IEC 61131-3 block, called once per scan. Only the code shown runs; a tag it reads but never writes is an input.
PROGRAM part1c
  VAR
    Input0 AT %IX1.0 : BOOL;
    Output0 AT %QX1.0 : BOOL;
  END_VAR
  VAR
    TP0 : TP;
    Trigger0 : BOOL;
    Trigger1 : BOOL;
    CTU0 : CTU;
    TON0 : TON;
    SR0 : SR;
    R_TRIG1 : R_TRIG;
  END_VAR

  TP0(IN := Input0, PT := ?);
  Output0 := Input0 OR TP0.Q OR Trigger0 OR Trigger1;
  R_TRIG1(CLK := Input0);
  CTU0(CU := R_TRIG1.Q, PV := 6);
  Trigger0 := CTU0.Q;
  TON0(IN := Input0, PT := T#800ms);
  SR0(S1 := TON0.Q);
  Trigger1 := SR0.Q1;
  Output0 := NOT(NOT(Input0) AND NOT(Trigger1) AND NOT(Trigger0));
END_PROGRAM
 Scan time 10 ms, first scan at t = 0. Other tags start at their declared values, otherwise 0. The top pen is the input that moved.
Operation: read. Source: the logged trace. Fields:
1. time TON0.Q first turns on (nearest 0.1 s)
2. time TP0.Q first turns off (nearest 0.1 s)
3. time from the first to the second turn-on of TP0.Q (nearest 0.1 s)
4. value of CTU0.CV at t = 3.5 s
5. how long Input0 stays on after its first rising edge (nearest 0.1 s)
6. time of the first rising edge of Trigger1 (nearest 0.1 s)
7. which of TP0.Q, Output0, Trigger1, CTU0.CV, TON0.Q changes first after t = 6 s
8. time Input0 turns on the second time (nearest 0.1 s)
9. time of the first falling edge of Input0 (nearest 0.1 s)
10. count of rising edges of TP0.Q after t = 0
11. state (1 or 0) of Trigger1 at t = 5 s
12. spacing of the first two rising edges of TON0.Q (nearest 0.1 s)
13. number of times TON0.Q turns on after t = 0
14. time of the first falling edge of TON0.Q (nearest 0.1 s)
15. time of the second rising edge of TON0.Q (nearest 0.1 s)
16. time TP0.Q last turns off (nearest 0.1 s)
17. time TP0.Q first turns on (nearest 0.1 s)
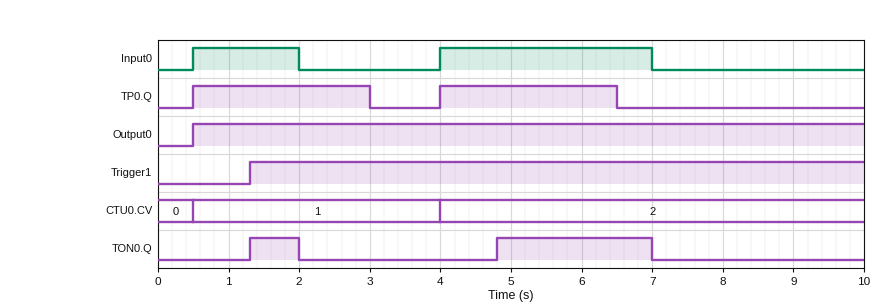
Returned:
1.3 s
3.0 s
3.5 s
1
1.5 s
1.3 s
TP0.Q
4.0 s
2.0 s
2
1
3.5 s
2
2.0 s
4.8 s
6.5 s
0.5 s
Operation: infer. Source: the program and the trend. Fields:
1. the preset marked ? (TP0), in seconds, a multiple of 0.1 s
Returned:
2.5 s
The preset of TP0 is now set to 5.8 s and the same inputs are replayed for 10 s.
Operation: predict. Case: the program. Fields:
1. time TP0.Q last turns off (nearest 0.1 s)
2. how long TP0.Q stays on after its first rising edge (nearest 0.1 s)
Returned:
6.3 s
5.8 s
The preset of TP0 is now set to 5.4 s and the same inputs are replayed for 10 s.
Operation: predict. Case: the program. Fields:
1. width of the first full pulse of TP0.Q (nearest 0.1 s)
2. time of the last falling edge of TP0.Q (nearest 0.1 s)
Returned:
5.4 s
5.9 s
